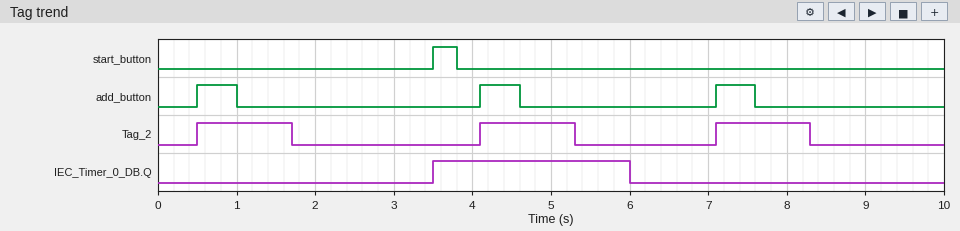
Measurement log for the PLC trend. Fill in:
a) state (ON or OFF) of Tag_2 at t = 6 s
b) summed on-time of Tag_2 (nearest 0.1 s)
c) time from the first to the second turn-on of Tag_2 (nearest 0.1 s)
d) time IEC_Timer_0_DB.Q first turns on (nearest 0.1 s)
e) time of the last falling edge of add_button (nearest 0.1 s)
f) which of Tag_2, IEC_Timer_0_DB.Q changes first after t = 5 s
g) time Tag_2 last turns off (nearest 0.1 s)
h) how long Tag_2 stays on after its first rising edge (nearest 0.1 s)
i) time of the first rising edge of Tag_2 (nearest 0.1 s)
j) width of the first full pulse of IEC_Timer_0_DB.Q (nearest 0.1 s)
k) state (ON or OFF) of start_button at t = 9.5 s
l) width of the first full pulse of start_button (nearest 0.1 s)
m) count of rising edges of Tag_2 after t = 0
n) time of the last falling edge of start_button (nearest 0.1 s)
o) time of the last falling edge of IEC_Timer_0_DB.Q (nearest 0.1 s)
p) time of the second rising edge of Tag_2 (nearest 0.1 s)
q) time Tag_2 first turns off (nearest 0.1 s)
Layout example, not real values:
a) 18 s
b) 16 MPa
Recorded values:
a) OFF
b) 3.6 s
c) 3.6 s
d) 3.5 s
e) 7.6 s
f) Tag_2
g) 8.3 s
h) 1.2 s
i) 0.5 s
j) 2.5 s
k) OFF
l) 0.3 s
m) 3
n) 3.8 s
o) 6.0 s
p) 4.1 s
q) 1.7 s
